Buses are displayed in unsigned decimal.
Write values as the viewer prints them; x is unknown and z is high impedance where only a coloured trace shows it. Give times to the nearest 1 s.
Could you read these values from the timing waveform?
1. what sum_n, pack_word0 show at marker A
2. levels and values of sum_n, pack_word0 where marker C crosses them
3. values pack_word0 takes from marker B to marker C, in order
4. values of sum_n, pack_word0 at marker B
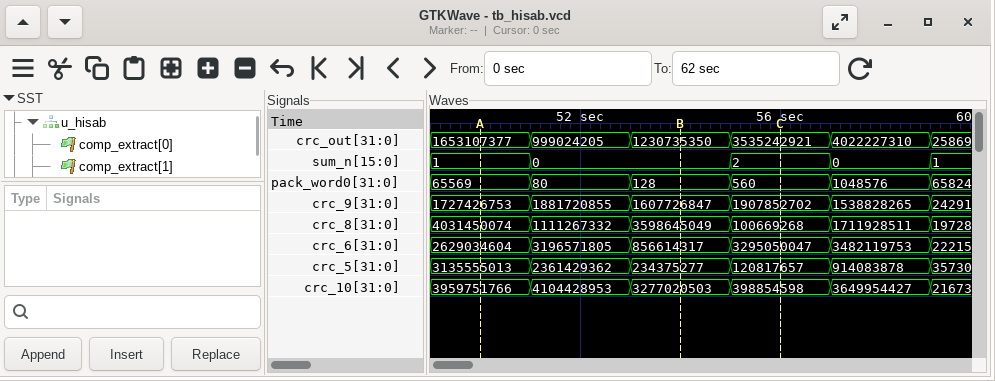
sum_n=1, pack_word0=65569
sum_n=2, pack_word0=560
128, 560
sum_n=0, pack_word0=128
